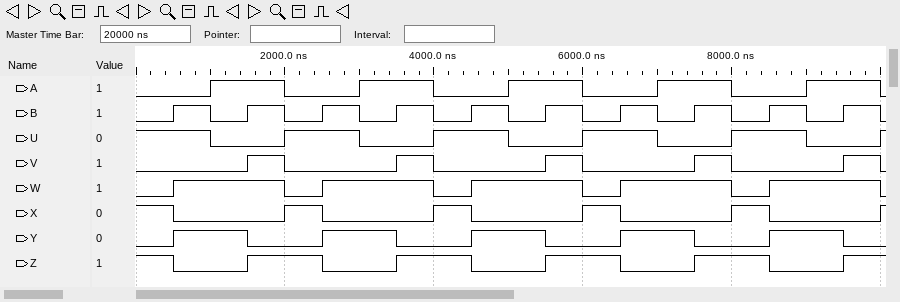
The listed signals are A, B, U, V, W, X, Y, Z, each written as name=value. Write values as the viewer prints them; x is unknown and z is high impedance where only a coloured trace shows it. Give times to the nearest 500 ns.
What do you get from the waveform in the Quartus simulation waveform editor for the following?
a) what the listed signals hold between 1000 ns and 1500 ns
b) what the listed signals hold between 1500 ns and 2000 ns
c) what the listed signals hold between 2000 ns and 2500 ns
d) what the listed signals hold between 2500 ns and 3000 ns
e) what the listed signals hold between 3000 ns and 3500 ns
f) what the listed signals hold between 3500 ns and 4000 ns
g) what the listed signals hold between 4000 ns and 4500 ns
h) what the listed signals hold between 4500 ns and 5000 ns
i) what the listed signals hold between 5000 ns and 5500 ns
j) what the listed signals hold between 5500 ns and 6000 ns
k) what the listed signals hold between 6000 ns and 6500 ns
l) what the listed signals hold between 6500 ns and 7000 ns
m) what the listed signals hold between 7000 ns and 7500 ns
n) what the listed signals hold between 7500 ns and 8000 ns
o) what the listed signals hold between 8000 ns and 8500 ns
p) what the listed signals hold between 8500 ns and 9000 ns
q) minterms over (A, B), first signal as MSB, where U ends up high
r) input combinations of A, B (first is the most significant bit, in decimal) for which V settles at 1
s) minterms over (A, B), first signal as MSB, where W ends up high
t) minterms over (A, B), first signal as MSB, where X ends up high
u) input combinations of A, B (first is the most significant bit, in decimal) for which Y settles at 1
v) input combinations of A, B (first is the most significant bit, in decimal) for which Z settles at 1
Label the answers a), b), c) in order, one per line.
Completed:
a) A=1, B=0, U=0, V=0, W=1, X=0, Y=1, Z=0
b) A=1, B=1, U=0, V=1, W=1, X=0, Y=0, Z=1
c) A=0, B=0, U=1, V=0, W=0, X=1, Y=0, Z=1
d) A=0, B=1, U=1, V=0, W=1, X=0, Y=1, Z=0
e) A=1, B=0, U=0, V=0, W=1, X=0, Y=1, Z=0
f) A=1, B=1, U=0, V=1, W=1, X=0, Y=0, Z=1
g) A=0, B=0, U=1, V=0, W=0, X=1, Y=0, Z=1
h) A=0, B=1, U=1, V=0, W=1, X=0, Y=1, Z=0
i) A=1, B=0, U=0, V=0, W=1, X=0, Y=1, Z=0
j) A=1, B=1, U=0, V=1, W=1, X=0, Y=0, Z=1
k) A=0, B=0, U=1, V=0, W=0, X=1, Y=0, Z=1
l) A=0, B=1, U=1, V=0, W=1, X=0, Y=1, Z=0
m) A=1, B=0, U=0, V=0, W=1, X=0, Y=1, Z=0
n) A=1, B=1, U=0, V=1, W=1, X=0, Y=0, Z=1
o) A=0, B=0, U=1, V=0, W=0, X=1, Y=0, Z=1
p) A=0, B=1, U=1, V=0, W=1, X=0, Y=1, Z=0
q) 0, 1
r) 3
s) 1, 2, 3
t) 0
u) 1, 2
v) 0, 3
